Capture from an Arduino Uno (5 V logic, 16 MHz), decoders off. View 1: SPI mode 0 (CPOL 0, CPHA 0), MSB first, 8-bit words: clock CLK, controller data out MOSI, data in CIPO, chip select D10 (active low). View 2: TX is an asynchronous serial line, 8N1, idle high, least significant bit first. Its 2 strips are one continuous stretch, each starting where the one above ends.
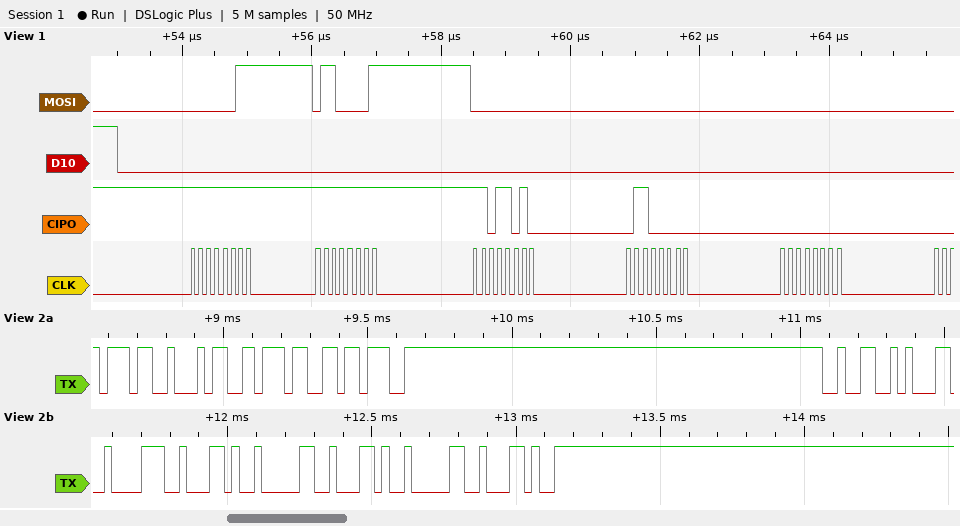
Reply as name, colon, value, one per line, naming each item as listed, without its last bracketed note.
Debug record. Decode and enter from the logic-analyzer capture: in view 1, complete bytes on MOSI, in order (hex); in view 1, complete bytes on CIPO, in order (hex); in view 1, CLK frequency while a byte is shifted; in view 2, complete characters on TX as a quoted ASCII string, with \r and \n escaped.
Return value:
in view 1, complete bytes on MOSI, in order: 03 61 00 00 00
in view 1, complete bytes on CIPO, in order: FF FF DA 60 00
in view 1, CLK frequency while a byte is shifted: 8 MHz
in view 2, complete characters on TX as a quoted ASCII string, with \r and \n escaped: "747;218,0,0,"
